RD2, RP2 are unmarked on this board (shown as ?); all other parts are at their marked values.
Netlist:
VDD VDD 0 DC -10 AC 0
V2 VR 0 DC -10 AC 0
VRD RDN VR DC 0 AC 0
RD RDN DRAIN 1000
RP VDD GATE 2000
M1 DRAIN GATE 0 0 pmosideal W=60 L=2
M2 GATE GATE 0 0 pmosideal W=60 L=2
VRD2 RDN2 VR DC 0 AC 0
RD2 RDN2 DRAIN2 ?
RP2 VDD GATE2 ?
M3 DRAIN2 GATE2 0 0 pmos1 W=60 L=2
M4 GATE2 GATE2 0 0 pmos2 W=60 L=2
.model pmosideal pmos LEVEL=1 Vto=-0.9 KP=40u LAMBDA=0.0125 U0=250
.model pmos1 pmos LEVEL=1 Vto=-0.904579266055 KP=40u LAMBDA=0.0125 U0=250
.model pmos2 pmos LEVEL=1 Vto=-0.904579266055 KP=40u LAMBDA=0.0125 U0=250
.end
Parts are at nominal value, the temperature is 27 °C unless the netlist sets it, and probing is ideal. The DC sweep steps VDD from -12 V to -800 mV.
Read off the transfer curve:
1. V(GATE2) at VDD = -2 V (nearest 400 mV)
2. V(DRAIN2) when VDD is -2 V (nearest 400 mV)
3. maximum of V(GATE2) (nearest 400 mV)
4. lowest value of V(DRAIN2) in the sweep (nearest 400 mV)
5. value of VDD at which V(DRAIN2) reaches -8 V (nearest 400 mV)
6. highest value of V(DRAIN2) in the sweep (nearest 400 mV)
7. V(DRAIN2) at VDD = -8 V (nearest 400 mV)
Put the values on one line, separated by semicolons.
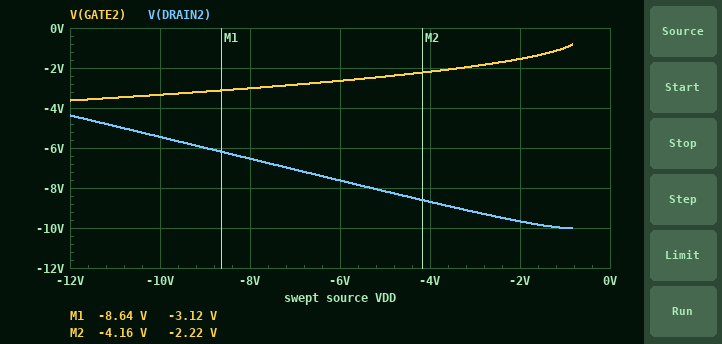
-1.6 V; -9.6 V; -800 mV; -10.0 V; -5.2 V; -4.4 V; -6.4 V
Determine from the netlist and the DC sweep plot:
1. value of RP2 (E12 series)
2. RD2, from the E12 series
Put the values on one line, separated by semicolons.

1.8 kΩ; 1.2 kΩ
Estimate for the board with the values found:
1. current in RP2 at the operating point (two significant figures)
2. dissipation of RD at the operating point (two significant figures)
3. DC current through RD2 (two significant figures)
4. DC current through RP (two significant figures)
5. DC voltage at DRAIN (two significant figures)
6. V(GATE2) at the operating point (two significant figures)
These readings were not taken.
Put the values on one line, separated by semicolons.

3.7 mA; 12 mW; 3.8 mA; 3.4 mA; -6.5 V; -3.3 V
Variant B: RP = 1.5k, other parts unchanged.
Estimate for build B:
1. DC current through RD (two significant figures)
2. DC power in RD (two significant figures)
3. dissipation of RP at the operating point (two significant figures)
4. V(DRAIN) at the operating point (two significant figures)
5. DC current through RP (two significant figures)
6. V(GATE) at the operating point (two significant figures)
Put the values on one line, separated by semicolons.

4.4 mA; 20 mW; 28 mW; -5.6 V; 4.3 mA; -3.5 V
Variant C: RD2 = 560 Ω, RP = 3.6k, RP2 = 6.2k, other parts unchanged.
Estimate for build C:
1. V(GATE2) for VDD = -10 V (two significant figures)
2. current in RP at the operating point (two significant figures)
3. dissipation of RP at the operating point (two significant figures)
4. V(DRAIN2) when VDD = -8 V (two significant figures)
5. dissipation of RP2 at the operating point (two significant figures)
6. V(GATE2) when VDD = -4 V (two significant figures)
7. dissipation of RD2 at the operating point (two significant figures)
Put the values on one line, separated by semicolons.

-2.3 V; 2.0 mA; 15 mW; -9.4 V; 9.5 mW; -1.7 V; 1.0 mW
